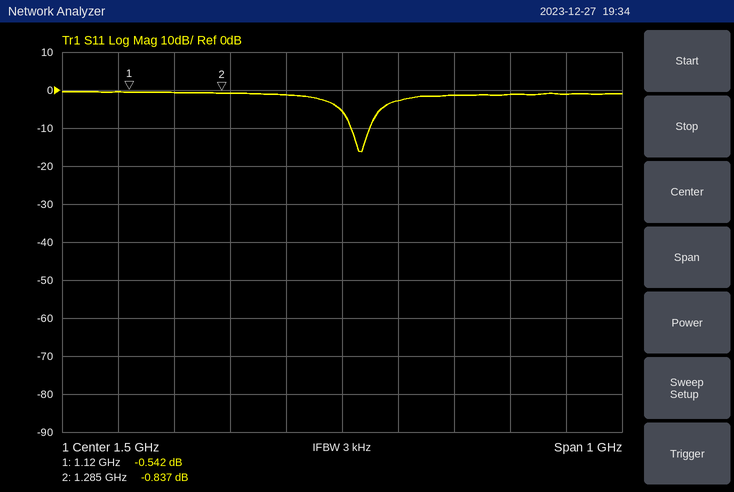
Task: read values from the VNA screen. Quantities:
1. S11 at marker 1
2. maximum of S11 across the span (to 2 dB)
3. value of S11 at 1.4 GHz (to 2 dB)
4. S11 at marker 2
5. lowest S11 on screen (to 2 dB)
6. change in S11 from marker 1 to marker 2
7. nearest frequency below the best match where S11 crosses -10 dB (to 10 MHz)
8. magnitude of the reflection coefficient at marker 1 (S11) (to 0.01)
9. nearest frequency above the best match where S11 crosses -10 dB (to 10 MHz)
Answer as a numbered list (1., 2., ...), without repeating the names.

1. -0.542 dB
2. 0 dB
3. -2 dB
4. -0.837 dB
5. -16 dB
6. -0.295 dB
7. 1.52 GHz
8. 0.94
9. 1.55 GHz
